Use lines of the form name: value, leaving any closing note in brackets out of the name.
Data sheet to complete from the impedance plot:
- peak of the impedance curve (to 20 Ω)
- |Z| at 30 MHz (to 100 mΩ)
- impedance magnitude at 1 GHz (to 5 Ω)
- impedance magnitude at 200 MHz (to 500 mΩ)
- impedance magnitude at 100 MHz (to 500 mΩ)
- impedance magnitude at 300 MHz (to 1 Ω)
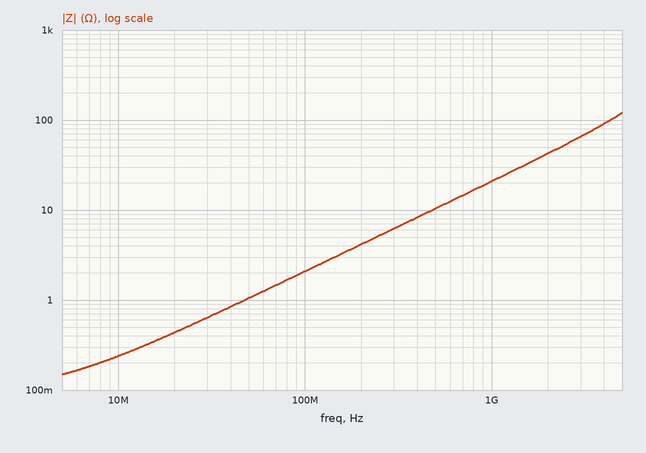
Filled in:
peak of the impedance curve: 120 Ω
|Z| at 30 MHz: 600 mΩ
impedance magnitude at 1 GHz: 20 Ω
impedance magnitude at 200 MHz: 4.0 Ω
impedance magnitude at 100 MHz: 2.0 Ω
impedance magnitude at 300 MHz: 6 Ω
